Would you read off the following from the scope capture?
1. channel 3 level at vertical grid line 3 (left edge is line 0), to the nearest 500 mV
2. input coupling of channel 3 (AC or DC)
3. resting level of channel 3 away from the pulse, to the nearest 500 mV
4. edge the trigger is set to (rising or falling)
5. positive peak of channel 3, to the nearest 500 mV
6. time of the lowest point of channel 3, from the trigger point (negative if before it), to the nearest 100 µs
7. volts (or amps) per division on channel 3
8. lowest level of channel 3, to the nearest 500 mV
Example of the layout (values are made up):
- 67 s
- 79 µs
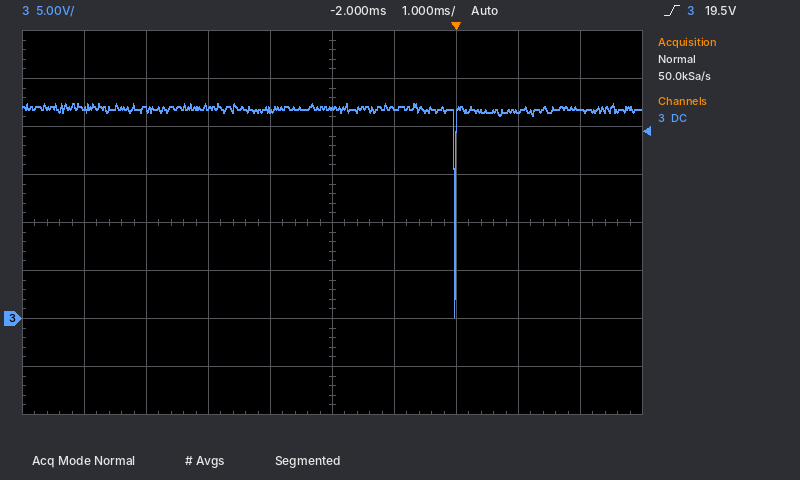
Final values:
- 22.0 V
- DC
- 22.0 V
- rising
- 22.5 V
- 0.0 ms
- 5 V
- 0.0 V
